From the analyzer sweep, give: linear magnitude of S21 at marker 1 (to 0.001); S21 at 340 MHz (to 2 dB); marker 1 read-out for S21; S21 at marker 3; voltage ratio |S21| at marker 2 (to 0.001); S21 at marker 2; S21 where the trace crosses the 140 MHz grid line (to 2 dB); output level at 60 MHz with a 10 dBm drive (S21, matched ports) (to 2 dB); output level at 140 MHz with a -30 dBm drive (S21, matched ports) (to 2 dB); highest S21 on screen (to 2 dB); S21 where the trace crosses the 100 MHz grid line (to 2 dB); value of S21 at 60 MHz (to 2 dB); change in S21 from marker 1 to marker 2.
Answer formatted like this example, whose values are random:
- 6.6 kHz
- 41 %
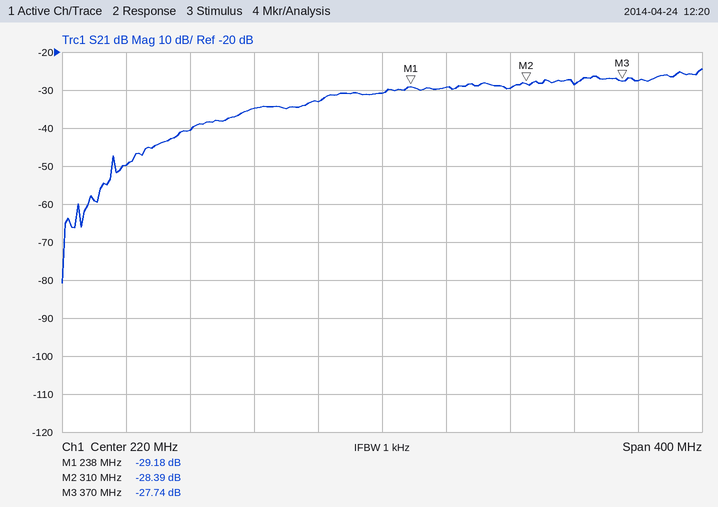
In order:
- 0.035
- -28 dB
- -29.18 dB
- -27.74 dB
- 0.038
- -28.39 dB
- -34 dB
- -40 dBm
- -64 dBm
- -24 dB
- -40 dB
- -50 dB
- 0.79 dB
